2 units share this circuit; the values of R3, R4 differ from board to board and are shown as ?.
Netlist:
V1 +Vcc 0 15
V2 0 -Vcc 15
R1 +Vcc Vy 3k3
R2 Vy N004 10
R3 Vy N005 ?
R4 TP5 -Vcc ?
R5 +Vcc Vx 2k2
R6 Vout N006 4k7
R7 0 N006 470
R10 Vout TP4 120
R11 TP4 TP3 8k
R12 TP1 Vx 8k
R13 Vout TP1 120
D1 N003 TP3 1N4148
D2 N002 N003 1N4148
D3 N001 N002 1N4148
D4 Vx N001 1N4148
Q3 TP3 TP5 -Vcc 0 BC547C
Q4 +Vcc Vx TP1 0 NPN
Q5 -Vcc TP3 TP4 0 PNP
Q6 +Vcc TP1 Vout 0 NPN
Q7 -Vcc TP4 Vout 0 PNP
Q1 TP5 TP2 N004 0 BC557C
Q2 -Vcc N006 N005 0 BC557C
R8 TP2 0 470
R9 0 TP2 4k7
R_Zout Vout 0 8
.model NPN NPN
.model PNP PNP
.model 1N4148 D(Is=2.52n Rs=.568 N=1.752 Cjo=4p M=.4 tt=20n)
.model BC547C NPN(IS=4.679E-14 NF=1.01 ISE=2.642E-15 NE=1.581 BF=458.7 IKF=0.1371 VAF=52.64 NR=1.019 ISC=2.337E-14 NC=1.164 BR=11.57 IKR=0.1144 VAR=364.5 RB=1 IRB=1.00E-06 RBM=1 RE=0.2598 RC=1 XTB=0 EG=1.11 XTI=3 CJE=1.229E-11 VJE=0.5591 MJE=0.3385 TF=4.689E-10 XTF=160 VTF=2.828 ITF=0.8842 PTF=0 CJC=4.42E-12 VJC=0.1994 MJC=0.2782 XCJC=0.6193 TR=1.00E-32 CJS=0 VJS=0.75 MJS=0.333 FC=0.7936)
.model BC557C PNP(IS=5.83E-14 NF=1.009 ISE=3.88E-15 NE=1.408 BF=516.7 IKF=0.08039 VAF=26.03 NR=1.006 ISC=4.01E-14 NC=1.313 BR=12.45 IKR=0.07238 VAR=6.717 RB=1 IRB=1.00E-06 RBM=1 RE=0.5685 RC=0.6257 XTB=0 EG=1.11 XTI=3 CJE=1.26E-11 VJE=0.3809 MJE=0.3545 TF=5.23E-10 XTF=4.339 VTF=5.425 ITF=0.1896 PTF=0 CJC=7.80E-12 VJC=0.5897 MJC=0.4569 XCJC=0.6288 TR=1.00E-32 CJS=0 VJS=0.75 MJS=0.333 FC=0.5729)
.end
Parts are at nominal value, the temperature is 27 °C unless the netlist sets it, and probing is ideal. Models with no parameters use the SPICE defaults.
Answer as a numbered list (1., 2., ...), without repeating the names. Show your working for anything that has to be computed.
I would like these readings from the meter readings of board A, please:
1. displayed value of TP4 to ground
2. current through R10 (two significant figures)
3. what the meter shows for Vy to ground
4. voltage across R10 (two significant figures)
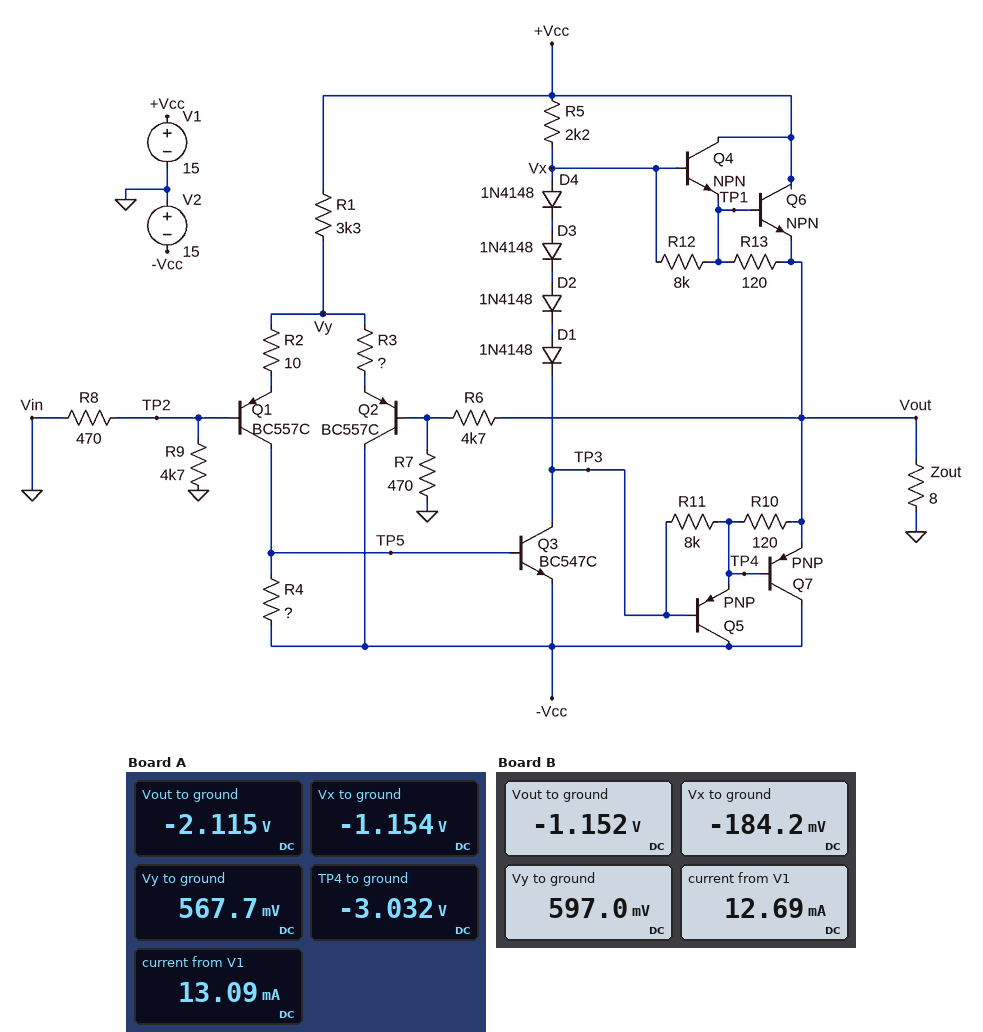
1. -3.032 V
2. (-2.115 V - (-3.032 V)) / 120 Ω = 7.6 mA
3. 567.7 mV
4. -2.115 V - (-3.032 V) = 920 mV
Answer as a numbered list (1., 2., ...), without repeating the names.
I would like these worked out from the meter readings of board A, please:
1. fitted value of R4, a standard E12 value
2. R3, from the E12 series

1. 3.3 kΩ
2. 27 Ω
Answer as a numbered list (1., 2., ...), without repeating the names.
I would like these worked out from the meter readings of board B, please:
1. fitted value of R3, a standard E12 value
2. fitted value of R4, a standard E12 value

1. 15 Ω
2. 1.2 kΩ
